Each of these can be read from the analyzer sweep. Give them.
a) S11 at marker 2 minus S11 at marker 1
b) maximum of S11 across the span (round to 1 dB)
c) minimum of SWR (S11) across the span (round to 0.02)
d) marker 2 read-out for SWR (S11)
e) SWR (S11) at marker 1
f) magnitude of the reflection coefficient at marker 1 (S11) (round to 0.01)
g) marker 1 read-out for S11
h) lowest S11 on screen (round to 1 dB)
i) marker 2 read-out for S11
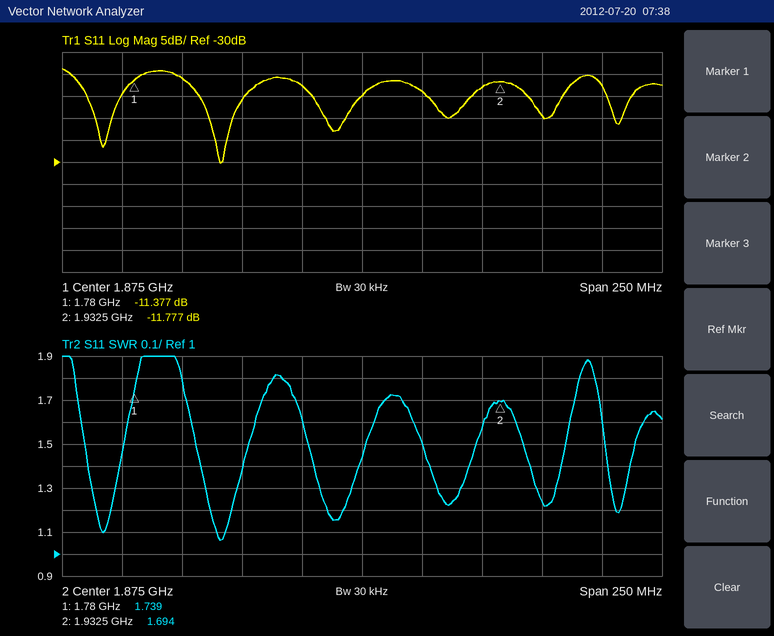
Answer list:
-0.400 dB
-9 dB
1.06
1.694
1.739
0.27
-11.377 dB
-30 dB
-11.777 dB
